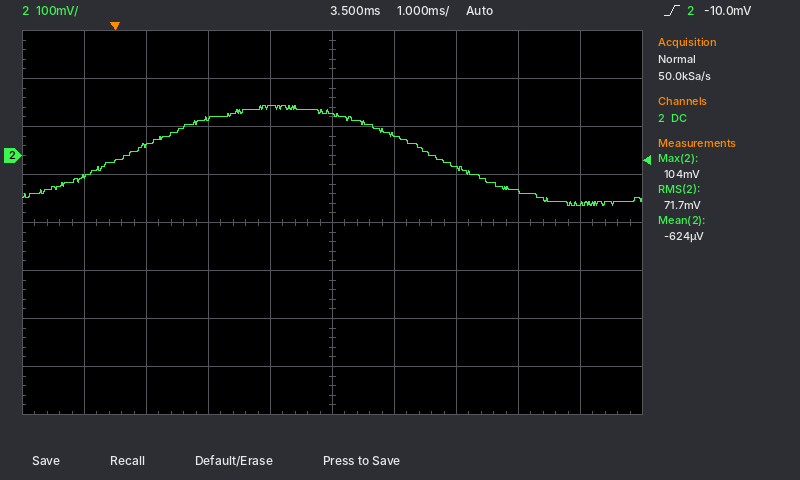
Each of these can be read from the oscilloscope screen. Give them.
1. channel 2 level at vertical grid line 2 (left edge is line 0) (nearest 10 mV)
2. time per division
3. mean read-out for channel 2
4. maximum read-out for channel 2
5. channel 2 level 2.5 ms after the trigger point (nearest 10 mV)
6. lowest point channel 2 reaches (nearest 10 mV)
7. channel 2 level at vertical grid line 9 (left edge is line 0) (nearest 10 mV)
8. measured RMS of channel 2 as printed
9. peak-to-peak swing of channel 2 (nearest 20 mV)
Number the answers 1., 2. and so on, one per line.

1. 20 mV
2. 1 ms
3. -624 µV
4. 104 mV
5. 100 mV
6. -100 mV
7. -100 mV
8. 71.7 mV
9. 200 mV
